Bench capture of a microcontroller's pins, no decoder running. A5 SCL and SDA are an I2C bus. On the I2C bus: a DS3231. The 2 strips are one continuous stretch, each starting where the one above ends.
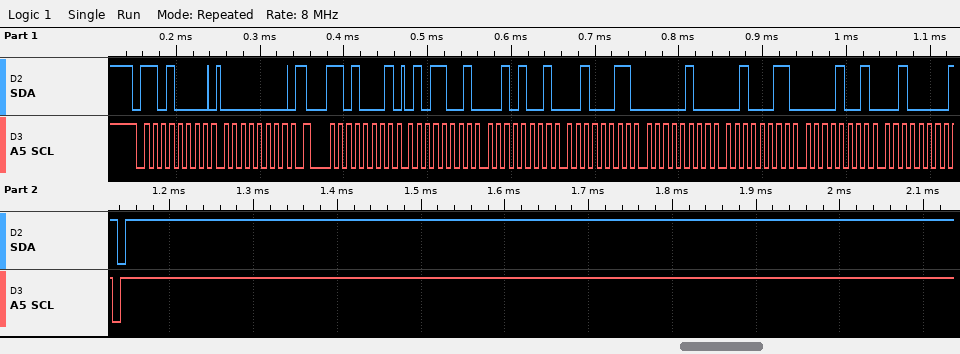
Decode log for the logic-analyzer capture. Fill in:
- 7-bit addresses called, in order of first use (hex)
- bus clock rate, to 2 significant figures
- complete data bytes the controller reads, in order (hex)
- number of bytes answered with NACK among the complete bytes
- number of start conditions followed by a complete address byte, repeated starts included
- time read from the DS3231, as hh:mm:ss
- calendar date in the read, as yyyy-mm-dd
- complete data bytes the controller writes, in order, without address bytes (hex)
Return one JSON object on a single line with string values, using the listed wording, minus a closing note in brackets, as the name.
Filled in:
{"7-bit addresses called, in order of first use": "0x68", "bus clock rate, to 2 significant figures": "100 kHz", "complete data bytes the controller reads, in order": "59 29 23 04 23 09 20", "number of bytes answered with NACK among the complete bytes": "1", "number of start conditions followed by a complete address byte, repeated starts included": "2", "time read from the DS3231, as hh:mm:ss": "23:29:59", "calendar date in the read, as yyyy-mm-dd": "2020-09-23", "complete data bytes the controller writes, in order, without address bytes": "00"}
